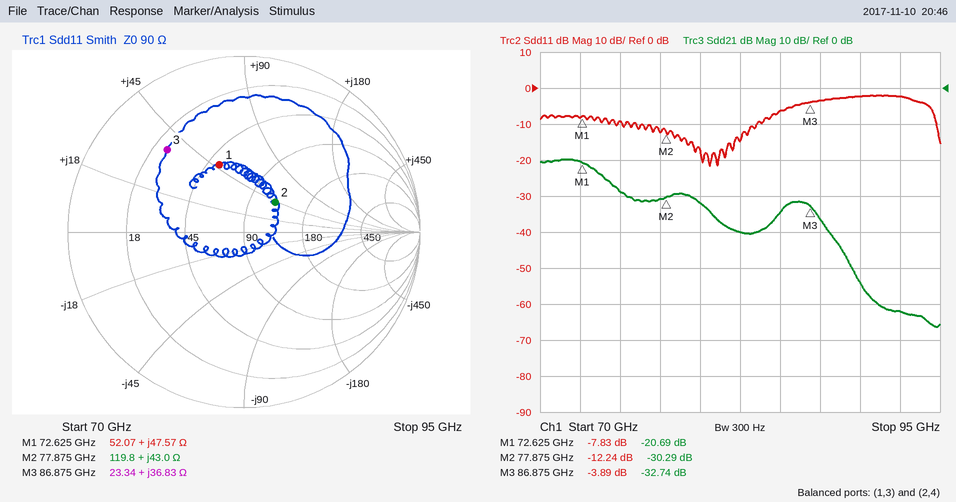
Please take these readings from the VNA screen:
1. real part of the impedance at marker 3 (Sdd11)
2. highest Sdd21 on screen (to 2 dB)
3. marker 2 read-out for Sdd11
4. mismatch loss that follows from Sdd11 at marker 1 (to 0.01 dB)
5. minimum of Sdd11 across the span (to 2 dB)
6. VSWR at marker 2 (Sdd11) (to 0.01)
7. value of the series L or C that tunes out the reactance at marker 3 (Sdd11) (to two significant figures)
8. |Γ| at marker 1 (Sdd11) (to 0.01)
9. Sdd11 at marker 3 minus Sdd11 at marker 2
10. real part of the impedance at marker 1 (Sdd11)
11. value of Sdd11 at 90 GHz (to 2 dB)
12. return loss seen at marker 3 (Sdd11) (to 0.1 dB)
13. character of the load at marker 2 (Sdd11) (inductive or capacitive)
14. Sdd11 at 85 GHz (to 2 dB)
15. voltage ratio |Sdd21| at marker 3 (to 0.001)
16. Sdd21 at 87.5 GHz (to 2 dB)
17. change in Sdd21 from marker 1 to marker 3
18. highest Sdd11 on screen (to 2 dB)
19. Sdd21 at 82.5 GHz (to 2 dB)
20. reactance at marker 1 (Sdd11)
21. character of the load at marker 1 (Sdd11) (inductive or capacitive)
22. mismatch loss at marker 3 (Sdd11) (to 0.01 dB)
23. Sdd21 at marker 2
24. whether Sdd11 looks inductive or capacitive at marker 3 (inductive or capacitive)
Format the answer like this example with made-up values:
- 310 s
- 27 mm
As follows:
- 23.34 Ω
- -20 dB
- -12.24 dB
- 0.78 dB
- -22 dB
- 1.65
- 50 fF
- 0.41
- 8.35 dB
- 52.07 Ω
- -2 dB
- 3.9 dB
- inductive
- -6 dB
- 0.023
- -36 dB
- -12.05 dB
- -2 dB
- -40 dB
- +47.57 Ω
- inductive
- 2.28 dB
- -30.29 dB
- inductive
